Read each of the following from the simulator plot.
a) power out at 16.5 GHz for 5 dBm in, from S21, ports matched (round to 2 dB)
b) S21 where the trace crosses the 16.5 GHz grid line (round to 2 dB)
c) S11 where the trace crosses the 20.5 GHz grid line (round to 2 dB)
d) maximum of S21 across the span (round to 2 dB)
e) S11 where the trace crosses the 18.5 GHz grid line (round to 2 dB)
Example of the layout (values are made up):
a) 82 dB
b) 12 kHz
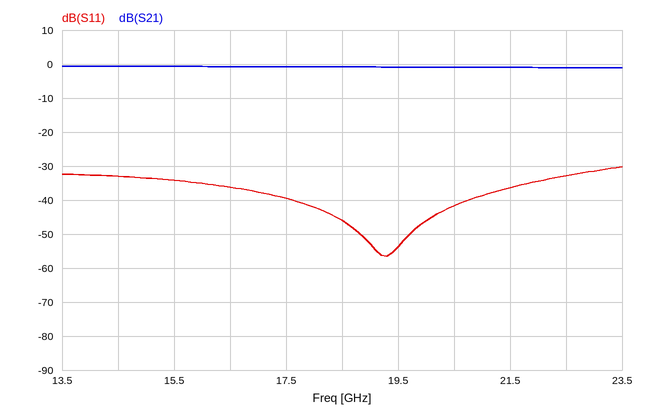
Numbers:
a) 4 dBm
b) 0 dB
c) -42 dB
d) 0 dB
e) -46 dB
